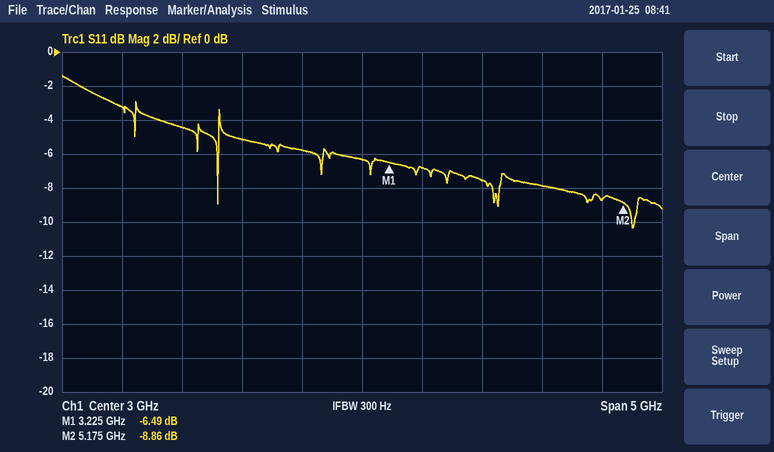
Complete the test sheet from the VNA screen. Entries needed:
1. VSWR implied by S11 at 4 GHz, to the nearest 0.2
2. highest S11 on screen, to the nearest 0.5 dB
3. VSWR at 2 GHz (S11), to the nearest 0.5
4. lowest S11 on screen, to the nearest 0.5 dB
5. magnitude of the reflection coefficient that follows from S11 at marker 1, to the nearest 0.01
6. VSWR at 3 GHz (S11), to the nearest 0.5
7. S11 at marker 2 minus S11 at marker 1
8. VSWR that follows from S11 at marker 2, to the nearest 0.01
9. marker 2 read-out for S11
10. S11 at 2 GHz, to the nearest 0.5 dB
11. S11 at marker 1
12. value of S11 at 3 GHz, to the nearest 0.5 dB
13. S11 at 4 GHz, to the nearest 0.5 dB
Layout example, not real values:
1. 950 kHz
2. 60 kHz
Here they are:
1. 2.4
2. -1.5 dB
3. 3.5
4. -10.5 dB
5. 0.47
6. 3.0
7. -2.37 dB
8. 2.13
9. -8.86 dB
10. -5.0 dB
11. -6.49 dB
12. -6.5 dB
13. -7.5 dB
